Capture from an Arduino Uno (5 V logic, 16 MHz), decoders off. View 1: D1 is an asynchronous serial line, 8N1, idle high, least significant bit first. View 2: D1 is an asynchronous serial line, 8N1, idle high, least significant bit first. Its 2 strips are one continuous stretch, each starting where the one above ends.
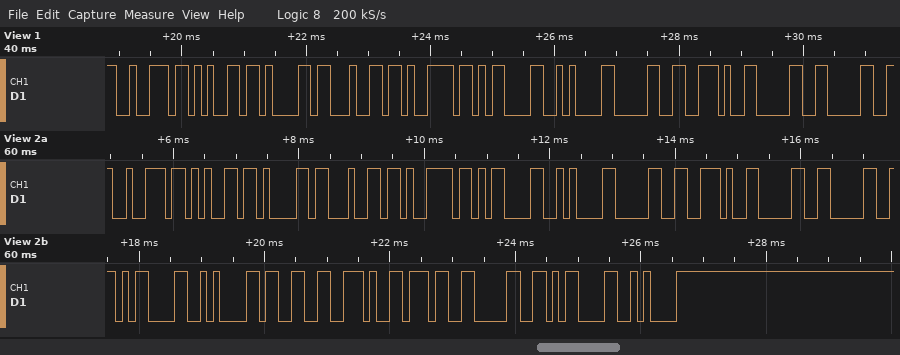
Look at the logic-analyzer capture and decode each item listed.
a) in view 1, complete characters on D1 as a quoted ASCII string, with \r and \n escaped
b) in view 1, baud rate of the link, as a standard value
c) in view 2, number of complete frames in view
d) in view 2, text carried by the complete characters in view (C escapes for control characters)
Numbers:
"ready\r\n0.00"
9600 baud
19
"ready\r\n0.00\r\n3.70\r\n"
